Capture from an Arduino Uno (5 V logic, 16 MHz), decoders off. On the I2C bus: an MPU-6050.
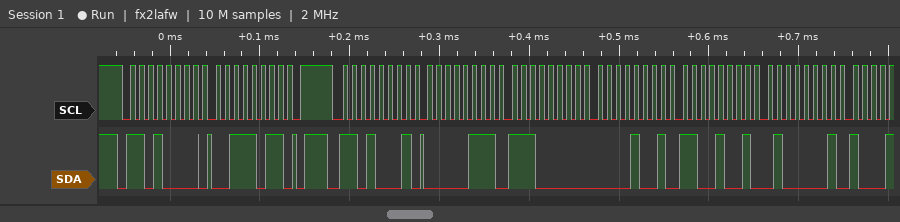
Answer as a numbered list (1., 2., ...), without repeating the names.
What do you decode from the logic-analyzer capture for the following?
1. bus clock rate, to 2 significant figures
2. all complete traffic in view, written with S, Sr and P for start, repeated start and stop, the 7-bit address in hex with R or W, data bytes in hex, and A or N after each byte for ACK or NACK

1. 100 kHz
2. S 68W A 3B A P S 68R A 07 A E0 A 09 A C9 A 41 A
